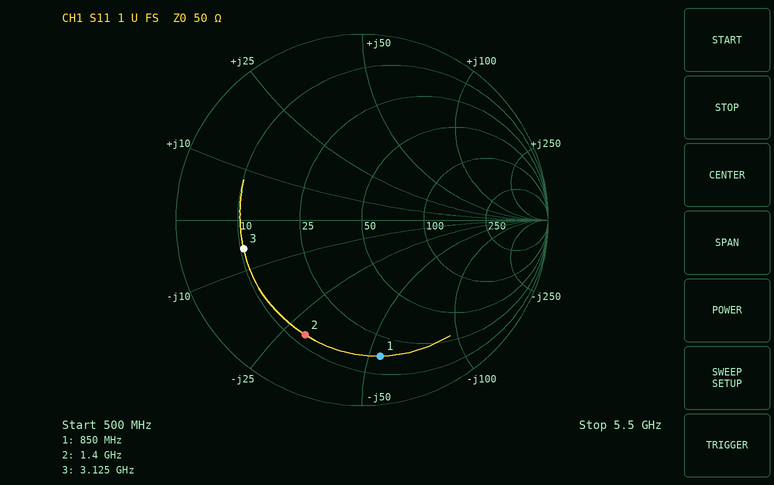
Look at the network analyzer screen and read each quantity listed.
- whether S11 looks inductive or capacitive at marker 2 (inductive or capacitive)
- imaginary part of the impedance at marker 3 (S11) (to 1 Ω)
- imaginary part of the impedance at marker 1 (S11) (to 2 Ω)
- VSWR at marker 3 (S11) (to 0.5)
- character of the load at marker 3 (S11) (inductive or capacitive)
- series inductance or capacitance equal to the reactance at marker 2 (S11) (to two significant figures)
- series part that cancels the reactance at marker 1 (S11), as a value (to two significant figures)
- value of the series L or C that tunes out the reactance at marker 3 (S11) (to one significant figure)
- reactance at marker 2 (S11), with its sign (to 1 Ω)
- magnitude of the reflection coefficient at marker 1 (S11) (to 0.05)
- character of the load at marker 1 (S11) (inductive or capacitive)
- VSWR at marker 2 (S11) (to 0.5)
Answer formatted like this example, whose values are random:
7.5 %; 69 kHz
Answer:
capacitive; -6 Ω; -54 Ω; 5.0; capacitive; 3.8 pF; 10 nH; 300 pH; -30 Ω; 0.75; capacitive; 5.5
